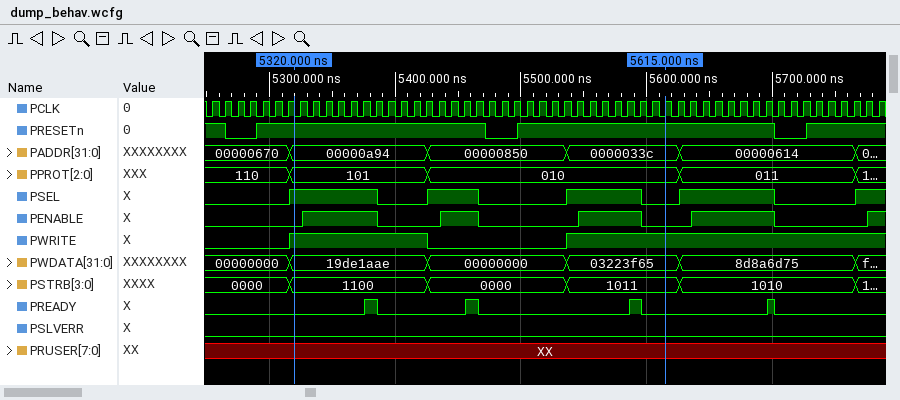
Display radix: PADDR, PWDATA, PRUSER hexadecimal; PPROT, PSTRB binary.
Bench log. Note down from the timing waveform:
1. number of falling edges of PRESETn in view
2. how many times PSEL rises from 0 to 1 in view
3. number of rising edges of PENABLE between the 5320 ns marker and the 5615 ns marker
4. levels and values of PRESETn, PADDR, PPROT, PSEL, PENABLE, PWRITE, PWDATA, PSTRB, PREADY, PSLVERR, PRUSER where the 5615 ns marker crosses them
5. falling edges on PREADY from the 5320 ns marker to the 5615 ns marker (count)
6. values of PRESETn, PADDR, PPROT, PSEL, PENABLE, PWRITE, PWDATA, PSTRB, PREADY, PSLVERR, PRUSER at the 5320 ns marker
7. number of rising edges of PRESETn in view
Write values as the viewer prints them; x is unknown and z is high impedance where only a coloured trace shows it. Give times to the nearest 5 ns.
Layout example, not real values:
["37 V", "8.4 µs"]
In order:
["3", "5", "3", "PRESETn=1, PADDR=0000033c, PPROT=010, PSEL=0, PENABLE=0, PWRITE=1, PWDATA=03223f65, PSTRB=1011, PREADY=0, PSLVERR=0, PRUSER=XX", "3", "PRESETn=1, PADDR=00000a94, PPROT=101, PSEL=1, PENABLE=0, PWRITE=1, PWDATA=19de1aae, PSTRB=1100, PREADY=0, PSLVERR=0, PRUSER=XX", "3"]
